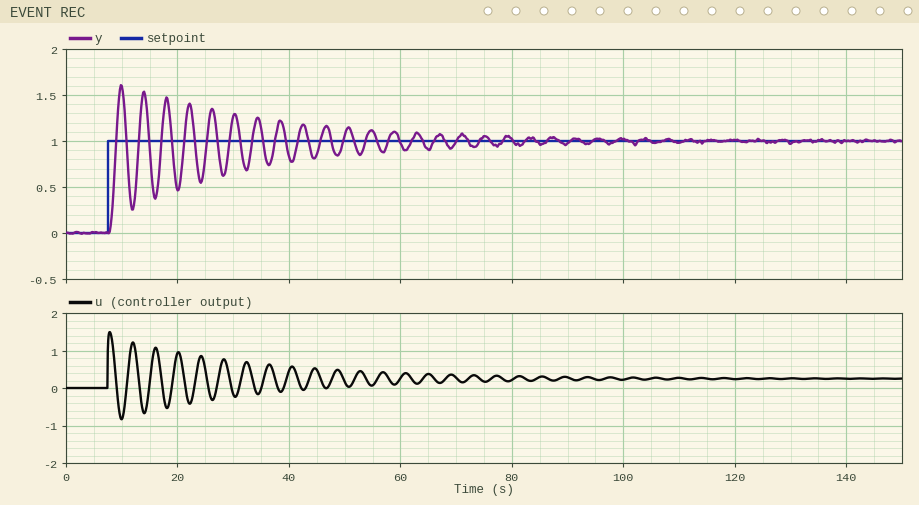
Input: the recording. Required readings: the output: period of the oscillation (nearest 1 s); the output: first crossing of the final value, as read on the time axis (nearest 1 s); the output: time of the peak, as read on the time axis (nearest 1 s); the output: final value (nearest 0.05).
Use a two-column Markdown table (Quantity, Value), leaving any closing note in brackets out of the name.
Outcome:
| Quantity | Value |
|---|---|
| the output: period of the oscillation | 4 s |
| the output: first crossing of the final value, as read on the time axis | 9 s |
| the output: time of the peak, as read on the time axis | 10 s |
| the output: final value | 1.00 |
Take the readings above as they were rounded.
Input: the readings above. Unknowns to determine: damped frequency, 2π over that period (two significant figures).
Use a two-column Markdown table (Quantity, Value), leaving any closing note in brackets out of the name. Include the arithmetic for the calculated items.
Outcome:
| Quantity | Value |
|---|---|
| damped frequency, 2π over that period | 2π / 4 = 1.6 rad/s |
